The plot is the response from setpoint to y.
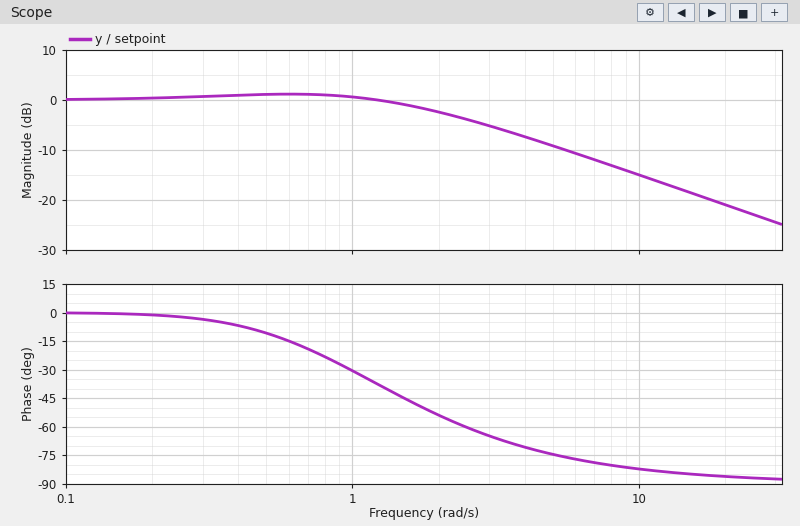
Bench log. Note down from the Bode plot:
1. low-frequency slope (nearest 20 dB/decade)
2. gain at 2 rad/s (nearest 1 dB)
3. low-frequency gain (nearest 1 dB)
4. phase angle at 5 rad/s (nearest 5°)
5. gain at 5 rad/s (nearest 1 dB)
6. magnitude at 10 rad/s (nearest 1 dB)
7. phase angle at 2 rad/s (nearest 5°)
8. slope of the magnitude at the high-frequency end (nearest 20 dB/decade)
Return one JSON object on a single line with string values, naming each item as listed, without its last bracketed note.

{"low-frequency slope": "0 dB/decade", "gain at 2 rad/s": "-2 dB", "low-frequency gain": "0 dB", "phase angle at 5 rad/s": "-75°", "gain at 5 rad/s": "-9 dB", "magnitude at 10 rad/s": "-15 dB", "phase angle at 2 rad/s": "-55°", "slope of the magnitude at the high-frequency end": "-20 dB/decade"}
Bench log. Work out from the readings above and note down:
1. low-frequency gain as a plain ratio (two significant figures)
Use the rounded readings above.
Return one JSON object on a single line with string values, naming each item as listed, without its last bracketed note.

{"low-frequency gain as a plain ratio": "1.0"}
